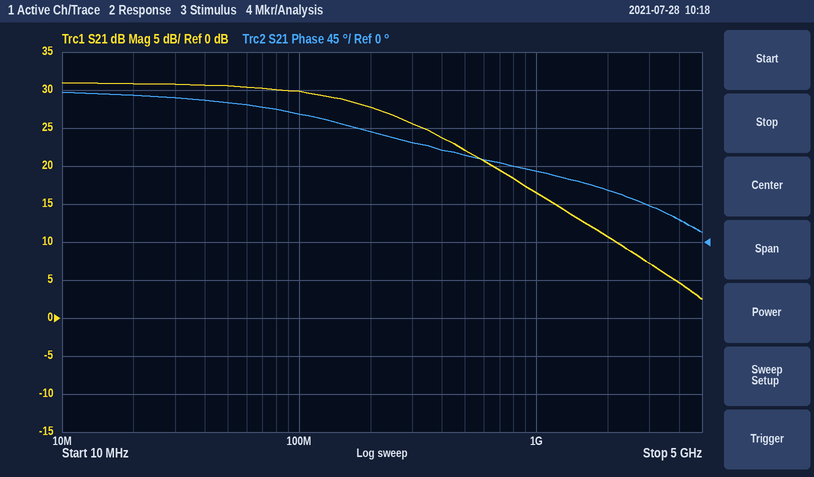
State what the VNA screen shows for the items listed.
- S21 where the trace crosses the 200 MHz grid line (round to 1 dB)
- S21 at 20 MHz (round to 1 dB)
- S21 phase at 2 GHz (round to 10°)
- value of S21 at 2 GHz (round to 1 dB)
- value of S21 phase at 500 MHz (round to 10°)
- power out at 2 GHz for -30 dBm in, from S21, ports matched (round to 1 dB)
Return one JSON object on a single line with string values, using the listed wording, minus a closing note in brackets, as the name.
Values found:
{"S21 where the trace crosses the 200 MHz grid line": "28 dB", "S21 at 20 MHz": "31 dB", "S21 phase at 2 GHz": "60°", "value of S21 at 2 GHz": "11 dB", "value of S21 phase at 500 MHz": "100°", "power out at 2 GHz for -30 dBm in, from S21, ports matched": "-19 dBm"}
